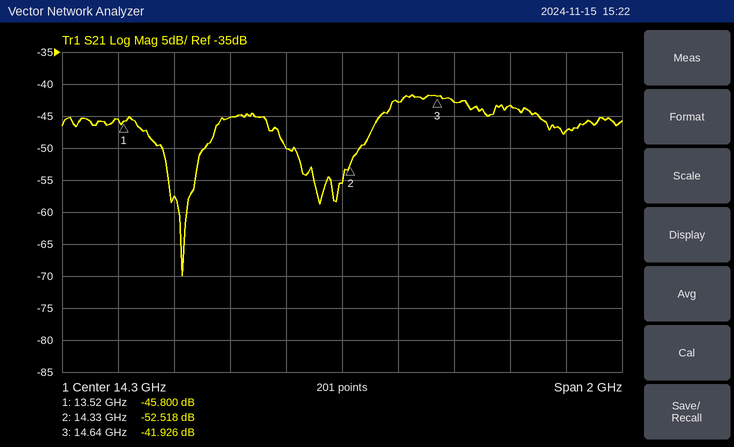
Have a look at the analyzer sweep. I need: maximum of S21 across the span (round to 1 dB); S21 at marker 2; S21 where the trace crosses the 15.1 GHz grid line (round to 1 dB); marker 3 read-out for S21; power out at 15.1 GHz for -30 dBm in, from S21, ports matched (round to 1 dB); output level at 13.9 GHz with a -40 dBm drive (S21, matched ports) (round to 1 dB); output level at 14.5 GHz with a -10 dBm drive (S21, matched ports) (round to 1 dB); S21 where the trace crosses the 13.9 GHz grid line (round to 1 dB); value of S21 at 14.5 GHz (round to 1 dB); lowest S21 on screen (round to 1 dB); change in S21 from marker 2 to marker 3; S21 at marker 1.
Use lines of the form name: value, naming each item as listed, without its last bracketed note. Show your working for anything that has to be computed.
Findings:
maximum of S21 across the span: -42 dB
S21 at marker 2: -52.518 dB
S21 where the trace crosses the 15.1 GHz grid line: -47 dB
marker 3 read-out for S21: -41.926 dB
power out at 15.1 GHz for -30 dBm in, from S21, ports matched: -30 dBm + (-47 dB) = -77 dBm
output level at 13.9 GHz with a -40 dBm drive (S21, matched ports): -40 dBm + (-45 dB) = -85 dBm
output level at 14.5 GHz with a -10 dBm drive (S21, matched ports): -10 dBm + (-43 dB) = -53 dBm
S21 where the trace crosses the 13.9 GHz grid line: -45 dB
value of S21 at 14.5 GHz: -43 dB
lowest S21 on screen: -70 dB
change in S21 from marker 2 to marker 3: -41.926 − (-52.518) = 10.592 dB
S21 at marker 1: -45.800 dB
